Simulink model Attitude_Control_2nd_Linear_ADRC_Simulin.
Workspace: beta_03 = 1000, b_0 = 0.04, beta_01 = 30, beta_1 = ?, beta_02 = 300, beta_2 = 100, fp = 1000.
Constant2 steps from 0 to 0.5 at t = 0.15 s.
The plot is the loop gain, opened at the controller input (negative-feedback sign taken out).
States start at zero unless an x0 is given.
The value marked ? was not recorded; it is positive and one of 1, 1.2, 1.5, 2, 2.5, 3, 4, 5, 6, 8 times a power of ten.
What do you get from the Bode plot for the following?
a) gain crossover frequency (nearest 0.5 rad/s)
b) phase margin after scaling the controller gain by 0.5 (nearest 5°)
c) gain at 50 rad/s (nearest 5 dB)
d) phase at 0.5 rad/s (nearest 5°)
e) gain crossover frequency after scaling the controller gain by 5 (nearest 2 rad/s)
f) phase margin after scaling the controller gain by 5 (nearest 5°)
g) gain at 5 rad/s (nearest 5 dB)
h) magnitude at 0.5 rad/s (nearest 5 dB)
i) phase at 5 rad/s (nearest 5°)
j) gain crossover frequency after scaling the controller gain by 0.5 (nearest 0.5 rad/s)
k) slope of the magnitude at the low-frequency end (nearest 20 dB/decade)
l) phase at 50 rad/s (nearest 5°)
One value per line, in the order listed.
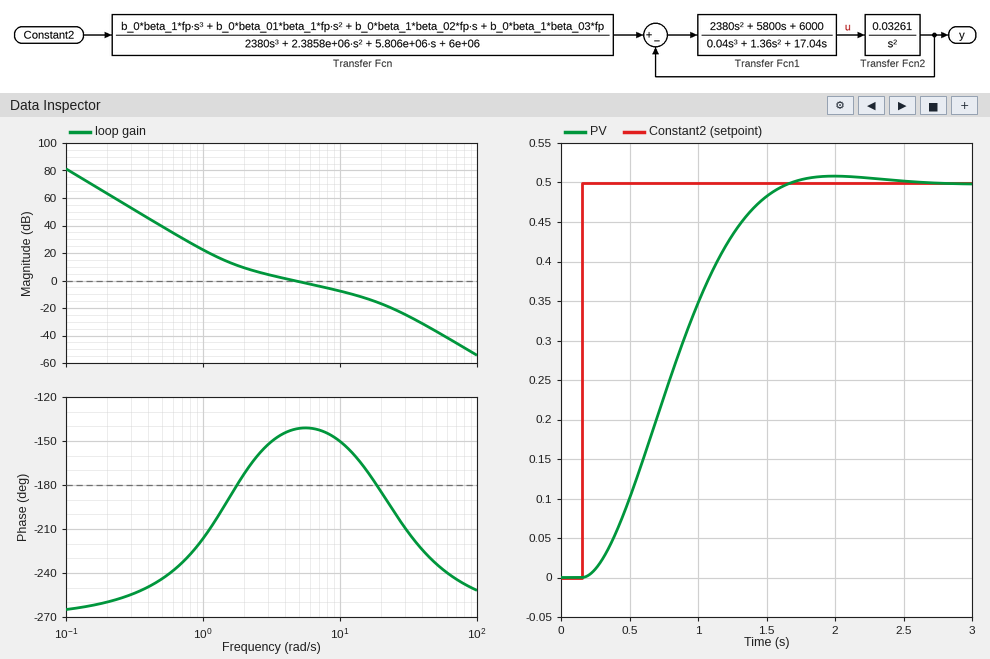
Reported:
4.5 rad/s
20°
-35 dB
-245°
16 rad/s
5°
0 dB
40 dB
-140°
2.5 rad/s
-60 dB/decade
-235°
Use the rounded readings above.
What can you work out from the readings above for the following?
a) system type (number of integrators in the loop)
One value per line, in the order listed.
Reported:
3
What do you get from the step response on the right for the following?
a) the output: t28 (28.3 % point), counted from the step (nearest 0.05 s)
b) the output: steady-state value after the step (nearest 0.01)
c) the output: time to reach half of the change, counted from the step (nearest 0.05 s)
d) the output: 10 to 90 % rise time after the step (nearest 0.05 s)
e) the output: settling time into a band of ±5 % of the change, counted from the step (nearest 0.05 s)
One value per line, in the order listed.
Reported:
0.45 s
0.50
0.65 s
0.95 s
1.30 s
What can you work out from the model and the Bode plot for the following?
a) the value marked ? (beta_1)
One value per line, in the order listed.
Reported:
150
